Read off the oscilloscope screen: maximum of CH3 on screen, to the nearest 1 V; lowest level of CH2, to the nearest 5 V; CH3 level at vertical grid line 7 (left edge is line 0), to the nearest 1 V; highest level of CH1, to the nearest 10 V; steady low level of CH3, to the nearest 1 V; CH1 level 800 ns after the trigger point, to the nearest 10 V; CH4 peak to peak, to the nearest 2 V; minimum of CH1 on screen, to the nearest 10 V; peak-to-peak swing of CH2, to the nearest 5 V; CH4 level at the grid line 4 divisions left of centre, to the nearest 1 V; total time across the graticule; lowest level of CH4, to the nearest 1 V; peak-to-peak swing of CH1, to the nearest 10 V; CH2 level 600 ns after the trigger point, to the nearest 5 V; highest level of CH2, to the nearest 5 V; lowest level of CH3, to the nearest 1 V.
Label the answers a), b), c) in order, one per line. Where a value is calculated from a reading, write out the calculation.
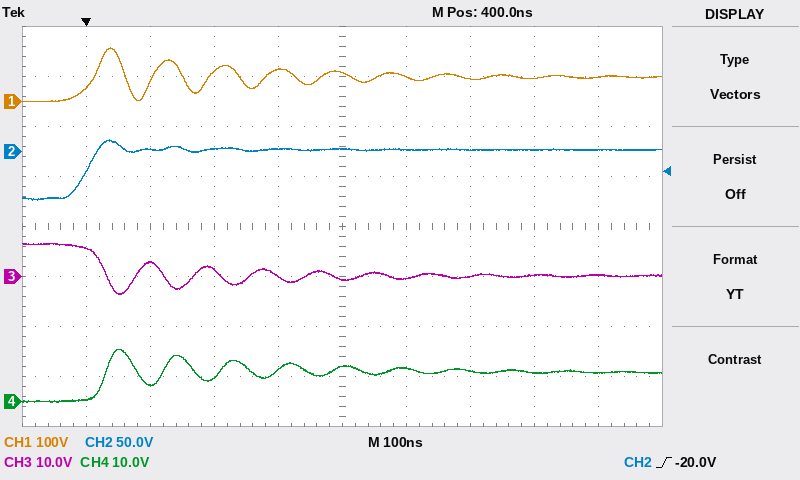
a) 7 V
b) -50 V
c) 0 V
d) 110 V
e) 0 V
f) 50 V
g) 10 V
h) 0 V
i) 10 V − (-50 V) = 60 V
j) 0 V
k) 1 µs
l) 0 V
m) 110 V − (0 V) = 110 V
n) 0 V
o) 10 V
p) -4 V
